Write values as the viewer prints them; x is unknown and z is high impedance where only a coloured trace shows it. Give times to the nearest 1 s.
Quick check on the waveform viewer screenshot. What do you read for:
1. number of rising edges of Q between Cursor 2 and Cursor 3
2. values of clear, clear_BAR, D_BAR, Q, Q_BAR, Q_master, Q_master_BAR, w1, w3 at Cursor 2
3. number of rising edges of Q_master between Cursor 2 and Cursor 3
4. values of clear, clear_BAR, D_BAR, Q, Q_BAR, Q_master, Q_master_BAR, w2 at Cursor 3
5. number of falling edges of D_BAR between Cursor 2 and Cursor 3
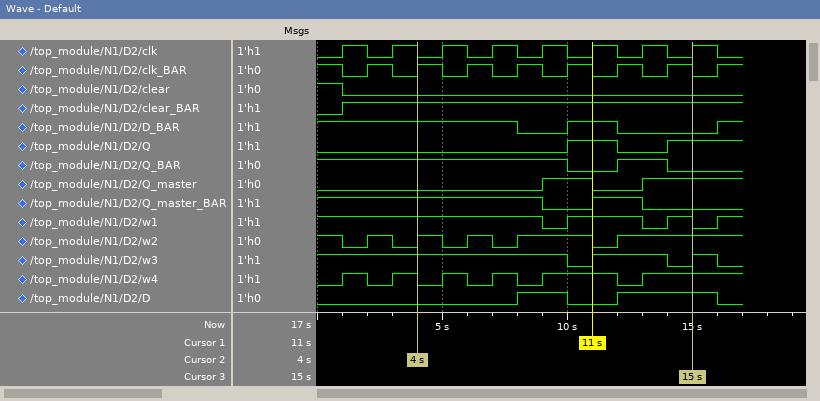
2
clear=0, clear_BAR=1, D_BAR=1, Q=0, Q_BAR=1, Q_master=0, Q_master_BAR=1, w1=1, w3=1
2
clear=0, clear_BAR=1, D_BAR=0, Q=1, Q_BAR=0, Q_master=1, Q_master_BAR=0, w2=1
2
